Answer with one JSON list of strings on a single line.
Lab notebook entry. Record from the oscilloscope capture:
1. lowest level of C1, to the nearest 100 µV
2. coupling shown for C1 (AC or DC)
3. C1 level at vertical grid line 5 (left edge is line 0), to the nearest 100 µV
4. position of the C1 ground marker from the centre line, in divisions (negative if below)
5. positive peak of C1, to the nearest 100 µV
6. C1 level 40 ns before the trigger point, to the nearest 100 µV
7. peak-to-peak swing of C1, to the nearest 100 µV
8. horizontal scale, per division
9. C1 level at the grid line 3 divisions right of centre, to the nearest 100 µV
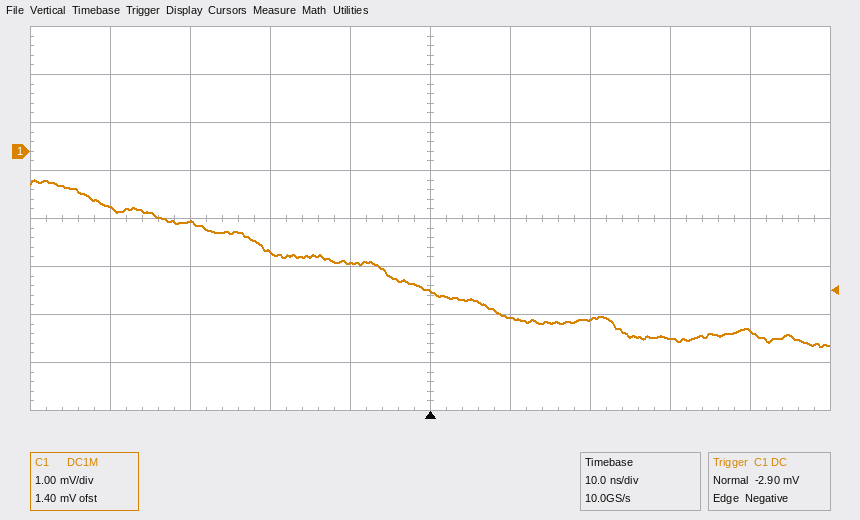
["-4.1 mV", "DC", "-2.9 mV", "+1.4 div", "-600 µV", "-1.2 mV", "3.5 mV", "10 ns", "-3.9 mV"]
